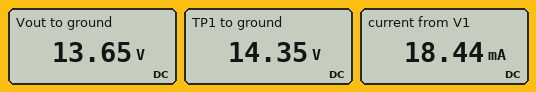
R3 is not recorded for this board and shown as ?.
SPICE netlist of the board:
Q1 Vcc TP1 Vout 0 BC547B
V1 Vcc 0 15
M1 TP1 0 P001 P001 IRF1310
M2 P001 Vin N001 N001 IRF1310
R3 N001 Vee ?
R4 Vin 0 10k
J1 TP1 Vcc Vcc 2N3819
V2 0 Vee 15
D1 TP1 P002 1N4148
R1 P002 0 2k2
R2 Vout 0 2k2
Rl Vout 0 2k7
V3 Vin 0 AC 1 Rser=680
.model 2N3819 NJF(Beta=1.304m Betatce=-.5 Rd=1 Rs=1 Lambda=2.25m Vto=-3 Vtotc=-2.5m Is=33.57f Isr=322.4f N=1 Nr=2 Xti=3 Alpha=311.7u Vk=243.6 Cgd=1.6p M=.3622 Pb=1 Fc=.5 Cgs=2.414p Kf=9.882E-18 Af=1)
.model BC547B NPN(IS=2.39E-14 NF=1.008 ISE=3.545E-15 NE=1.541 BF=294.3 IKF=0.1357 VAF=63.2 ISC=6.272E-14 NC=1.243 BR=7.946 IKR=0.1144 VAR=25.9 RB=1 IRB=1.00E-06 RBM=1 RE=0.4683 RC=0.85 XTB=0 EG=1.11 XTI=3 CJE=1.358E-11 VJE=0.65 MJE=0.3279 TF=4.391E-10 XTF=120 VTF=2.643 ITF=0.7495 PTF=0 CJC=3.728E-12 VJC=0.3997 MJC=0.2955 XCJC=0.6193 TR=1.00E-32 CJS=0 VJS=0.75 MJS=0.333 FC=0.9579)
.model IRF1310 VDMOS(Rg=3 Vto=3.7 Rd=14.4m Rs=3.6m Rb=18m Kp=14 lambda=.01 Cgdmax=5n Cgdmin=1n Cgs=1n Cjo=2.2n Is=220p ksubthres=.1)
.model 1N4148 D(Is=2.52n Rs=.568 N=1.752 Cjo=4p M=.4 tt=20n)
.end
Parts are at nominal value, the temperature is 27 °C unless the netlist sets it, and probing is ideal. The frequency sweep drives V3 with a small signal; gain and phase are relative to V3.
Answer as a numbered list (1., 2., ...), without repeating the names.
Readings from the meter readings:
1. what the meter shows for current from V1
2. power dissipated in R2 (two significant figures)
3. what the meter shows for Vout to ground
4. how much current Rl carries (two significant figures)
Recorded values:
1. 18.44 mA
2. 85 mW
3. 13.65 V
4. 5.1 mA
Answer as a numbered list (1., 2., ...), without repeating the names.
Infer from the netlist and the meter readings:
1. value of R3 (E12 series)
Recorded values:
1. 12 kΩ
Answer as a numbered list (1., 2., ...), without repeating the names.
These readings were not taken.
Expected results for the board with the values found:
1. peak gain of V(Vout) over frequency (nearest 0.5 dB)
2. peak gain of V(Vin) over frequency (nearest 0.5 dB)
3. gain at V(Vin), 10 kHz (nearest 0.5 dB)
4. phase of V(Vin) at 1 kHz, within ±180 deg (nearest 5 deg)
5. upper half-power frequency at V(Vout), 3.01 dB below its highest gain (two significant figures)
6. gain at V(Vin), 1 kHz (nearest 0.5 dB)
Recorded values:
1. -34.5 dB
2. -0.5 dB
3. -1.0 dB
4. 0 deg
5. 2.2 MHz
6. -0.5 dB
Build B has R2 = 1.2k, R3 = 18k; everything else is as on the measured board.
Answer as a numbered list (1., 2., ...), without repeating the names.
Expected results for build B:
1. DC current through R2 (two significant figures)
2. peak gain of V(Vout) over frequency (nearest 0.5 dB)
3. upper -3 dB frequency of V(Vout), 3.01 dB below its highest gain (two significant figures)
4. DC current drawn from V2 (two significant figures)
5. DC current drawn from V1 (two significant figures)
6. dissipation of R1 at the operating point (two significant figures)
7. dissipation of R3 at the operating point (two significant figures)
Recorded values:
1. 11 mA
2. -34.0 dB
3. 1.7 MHz
4. 640 µA
5. 23 mA
6. 85 mW
7. 7.4 mW
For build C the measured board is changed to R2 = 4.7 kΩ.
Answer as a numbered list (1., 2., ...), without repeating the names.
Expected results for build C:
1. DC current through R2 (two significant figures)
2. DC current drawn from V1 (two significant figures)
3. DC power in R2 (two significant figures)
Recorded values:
1. 2.9 mA
2. 15 mA
3. 40 mW
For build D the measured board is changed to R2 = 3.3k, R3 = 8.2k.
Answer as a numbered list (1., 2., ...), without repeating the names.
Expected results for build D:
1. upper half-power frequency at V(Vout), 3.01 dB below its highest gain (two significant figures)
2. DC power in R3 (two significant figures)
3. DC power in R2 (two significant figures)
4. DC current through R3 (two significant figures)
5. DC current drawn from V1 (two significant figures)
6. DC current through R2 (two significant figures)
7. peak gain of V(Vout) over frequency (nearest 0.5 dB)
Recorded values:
1. 3.0 MHz
2. 16 mW
3. 56 mW
4. 1.4 mA
5. 17 mA
6. 4.1 mA
7. -36.0 dB
